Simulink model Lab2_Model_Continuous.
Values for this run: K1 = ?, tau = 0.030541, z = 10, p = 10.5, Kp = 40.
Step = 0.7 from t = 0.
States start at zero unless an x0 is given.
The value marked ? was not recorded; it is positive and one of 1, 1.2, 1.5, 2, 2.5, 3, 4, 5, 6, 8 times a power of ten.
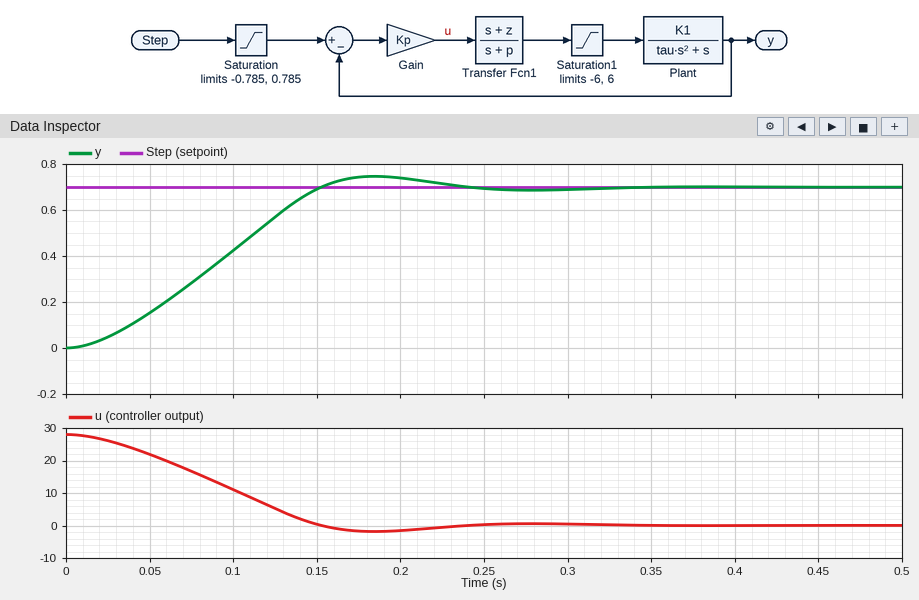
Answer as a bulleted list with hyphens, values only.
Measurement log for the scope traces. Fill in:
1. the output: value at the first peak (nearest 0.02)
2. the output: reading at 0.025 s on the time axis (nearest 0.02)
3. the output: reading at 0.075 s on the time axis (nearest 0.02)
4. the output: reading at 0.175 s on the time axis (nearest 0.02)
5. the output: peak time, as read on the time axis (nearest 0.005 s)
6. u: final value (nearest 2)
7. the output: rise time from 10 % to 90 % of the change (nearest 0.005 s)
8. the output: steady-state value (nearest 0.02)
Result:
- 0.74
- 0.04
- 0.28
- 0.74
- 0.185 s
- 0
- 0.105 s
- 0.70
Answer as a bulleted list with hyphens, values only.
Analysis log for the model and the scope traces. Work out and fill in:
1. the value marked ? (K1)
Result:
- 1
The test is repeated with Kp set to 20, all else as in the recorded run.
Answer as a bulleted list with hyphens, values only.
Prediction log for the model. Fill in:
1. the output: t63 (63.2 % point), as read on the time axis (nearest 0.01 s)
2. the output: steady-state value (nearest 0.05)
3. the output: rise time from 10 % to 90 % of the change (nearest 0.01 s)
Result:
- 0.10 s
- 0.70
- 0.11 s
